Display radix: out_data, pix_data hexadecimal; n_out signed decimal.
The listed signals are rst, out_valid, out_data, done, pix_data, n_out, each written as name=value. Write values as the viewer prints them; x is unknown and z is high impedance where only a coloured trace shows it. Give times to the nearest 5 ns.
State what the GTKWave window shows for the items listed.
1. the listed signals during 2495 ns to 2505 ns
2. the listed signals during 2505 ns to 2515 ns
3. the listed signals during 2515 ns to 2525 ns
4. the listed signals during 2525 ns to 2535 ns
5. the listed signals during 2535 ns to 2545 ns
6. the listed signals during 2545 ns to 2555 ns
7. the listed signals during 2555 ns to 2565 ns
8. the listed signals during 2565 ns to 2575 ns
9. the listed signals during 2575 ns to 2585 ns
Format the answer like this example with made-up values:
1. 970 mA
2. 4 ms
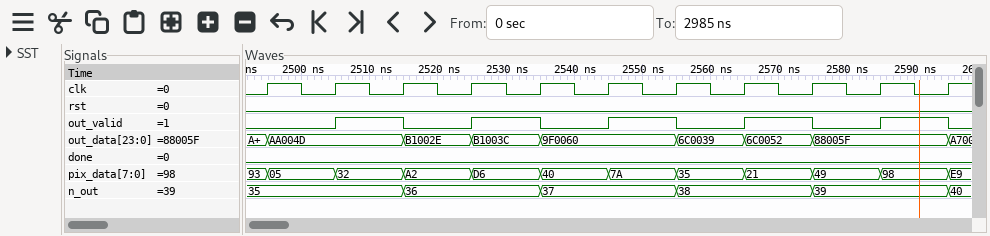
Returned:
1. rst=0, out_valid=0, out_data=AA004D, done=0, pix_data=05, n_out=35
2. rst=0, out_valid=1, out_data=AA004D, done=0, pix_data=32, n_out=35
3. rst=0, out_valid=0, out_data=B1002E, done=0, pix_data=A2, n_out=36
4. rst=0, out_valid=1, out_data=B1003C, done=0, pix_data=D6, n_out=36
5. rst=0, out_valid=0, out_data=9F0060, done=0, pix_data=40, n_out=37
6. rst=0, out_valid=1, out_data=9F0060, done=0, pix_data=7A, n_out=37
7. rst=0, out_valid=0, out_data=6C0039, done=0, pix_data=35, n_out=38
8. rst=0, out_valid=1, out_data=6C0052, done=0, pix_data=21, n_out=38
9. rst=0, out_valid=0, out_data=88005F, done=0, pix_data=49, n_out=39
